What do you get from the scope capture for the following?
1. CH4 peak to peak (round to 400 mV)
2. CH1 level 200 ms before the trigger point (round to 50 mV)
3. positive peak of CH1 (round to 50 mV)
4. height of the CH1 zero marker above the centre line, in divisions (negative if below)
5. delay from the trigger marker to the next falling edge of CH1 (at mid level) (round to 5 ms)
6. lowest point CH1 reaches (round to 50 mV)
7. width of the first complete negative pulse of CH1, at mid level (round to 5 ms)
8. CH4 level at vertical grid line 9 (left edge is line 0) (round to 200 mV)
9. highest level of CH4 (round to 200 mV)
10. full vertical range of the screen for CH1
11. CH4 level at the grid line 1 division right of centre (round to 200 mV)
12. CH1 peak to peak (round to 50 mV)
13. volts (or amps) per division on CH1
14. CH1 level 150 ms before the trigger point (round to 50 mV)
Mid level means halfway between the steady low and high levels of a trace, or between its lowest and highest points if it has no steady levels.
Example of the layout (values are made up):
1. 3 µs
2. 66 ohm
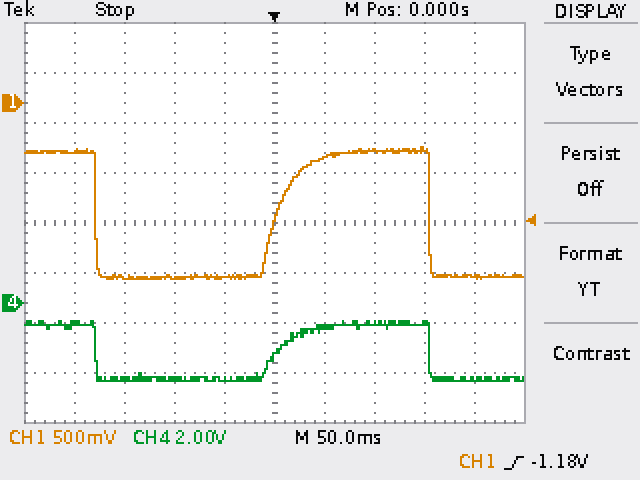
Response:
1. 2.4 V
2. -500 mV
3. -450 mV
4. +2.4 div
5. 155 ms
6. -1.75 V
7. 180 ms
8. -3.0 V
9. -800 mV
10. 4 V
11. -1.0 V
12. 1.30 V
13. 500 mV
14. -1.75 V
